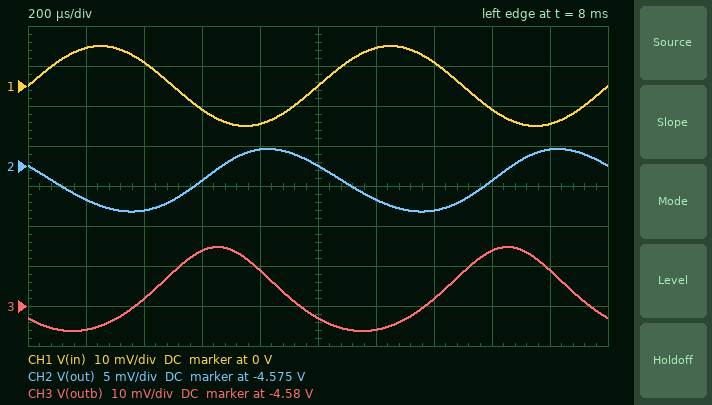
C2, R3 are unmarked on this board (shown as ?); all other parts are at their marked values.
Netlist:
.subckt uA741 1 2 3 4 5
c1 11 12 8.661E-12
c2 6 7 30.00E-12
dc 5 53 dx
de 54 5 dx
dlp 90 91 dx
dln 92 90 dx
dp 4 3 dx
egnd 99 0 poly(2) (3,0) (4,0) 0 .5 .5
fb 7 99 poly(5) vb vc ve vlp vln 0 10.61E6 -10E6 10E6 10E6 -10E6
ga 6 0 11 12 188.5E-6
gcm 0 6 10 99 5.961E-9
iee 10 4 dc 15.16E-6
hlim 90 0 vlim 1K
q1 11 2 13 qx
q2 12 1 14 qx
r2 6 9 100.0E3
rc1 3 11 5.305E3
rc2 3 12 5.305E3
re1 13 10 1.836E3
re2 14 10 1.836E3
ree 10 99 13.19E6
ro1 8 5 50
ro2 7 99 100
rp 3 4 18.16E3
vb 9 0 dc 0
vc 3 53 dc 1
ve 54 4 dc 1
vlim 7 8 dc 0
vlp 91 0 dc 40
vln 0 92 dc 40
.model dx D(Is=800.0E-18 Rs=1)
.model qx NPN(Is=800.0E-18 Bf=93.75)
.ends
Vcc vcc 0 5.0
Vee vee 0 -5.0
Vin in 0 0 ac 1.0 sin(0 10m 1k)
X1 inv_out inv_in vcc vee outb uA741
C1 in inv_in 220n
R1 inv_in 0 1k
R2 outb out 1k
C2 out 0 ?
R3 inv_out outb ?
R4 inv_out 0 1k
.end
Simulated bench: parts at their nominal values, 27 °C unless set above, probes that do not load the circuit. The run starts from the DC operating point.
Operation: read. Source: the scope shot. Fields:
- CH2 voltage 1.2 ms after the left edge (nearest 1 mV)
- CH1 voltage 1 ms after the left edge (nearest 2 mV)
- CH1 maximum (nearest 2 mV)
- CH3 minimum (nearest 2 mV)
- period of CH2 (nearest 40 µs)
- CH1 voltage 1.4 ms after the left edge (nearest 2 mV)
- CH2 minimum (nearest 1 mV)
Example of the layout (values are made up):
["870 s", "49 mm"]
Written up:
["-4.579 V", "0 V", "10 mV", "-4.586 V", "1.00 ms", "6 mV", "-4.581 V"]
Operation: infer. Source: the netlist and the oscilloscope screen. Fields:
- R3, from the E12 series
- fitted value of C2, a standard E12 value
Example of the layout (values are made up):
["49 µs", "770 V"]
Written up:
["220 kΩ", "390 nF"]
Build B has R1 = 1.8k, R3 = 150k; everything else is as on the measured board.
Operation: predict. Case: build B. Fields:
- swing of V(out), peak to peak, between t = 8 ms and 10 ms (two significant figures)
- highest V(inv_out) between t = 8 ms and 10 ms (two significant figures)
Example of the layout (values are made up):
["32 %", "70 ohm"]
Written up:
["5.8 mV", "-30 mV"]
